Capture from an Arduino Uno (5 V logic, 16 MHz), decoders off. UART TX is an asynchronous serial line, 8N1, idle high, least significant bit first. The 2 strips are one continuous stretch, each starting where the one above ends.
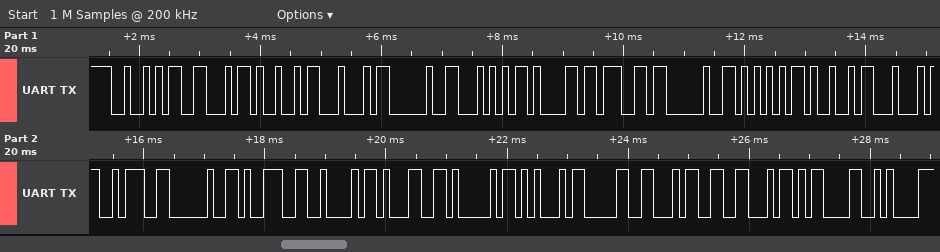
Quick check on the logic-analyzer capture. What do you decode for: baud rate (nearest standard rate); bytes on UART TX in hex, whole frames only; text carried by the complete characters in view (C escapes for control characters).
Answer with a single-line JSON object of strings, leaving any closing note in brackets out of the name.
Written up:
{"baud rate": "9600 baud", "bytes on UART TX in hex, whole frames only": "52 46 49 44 20 54 61 67 20 55 49 44 3A 20 39 42 31 41 45 30 34 46 0D 0A", "text carried by the complete characters in view": "\"RFID Tag UID: 9B1AE04F\\r\\n\""}
